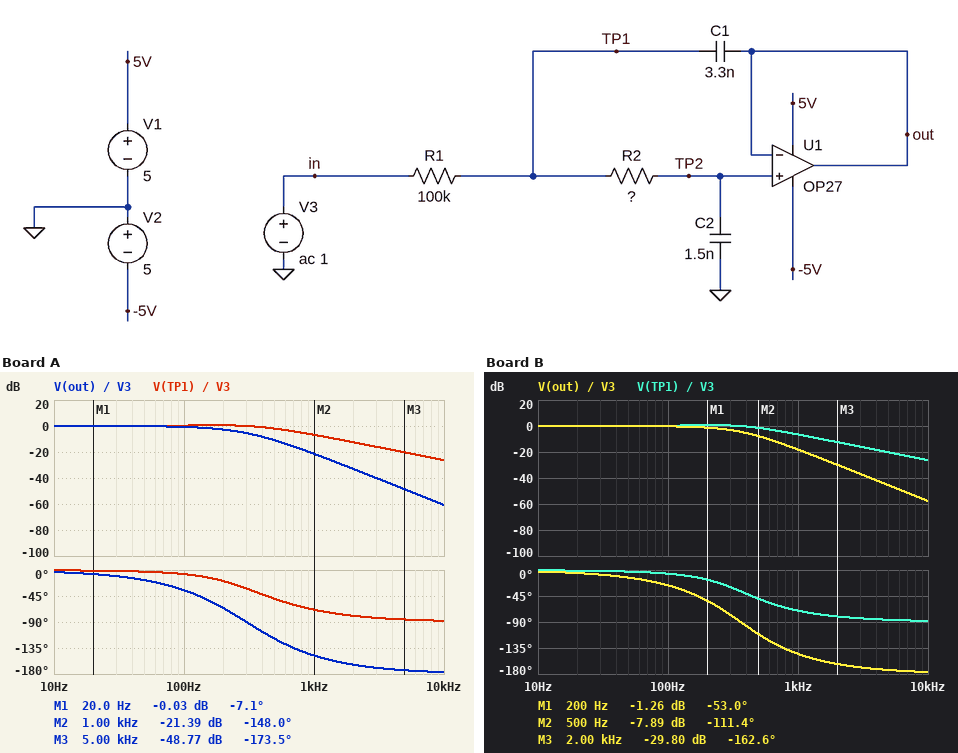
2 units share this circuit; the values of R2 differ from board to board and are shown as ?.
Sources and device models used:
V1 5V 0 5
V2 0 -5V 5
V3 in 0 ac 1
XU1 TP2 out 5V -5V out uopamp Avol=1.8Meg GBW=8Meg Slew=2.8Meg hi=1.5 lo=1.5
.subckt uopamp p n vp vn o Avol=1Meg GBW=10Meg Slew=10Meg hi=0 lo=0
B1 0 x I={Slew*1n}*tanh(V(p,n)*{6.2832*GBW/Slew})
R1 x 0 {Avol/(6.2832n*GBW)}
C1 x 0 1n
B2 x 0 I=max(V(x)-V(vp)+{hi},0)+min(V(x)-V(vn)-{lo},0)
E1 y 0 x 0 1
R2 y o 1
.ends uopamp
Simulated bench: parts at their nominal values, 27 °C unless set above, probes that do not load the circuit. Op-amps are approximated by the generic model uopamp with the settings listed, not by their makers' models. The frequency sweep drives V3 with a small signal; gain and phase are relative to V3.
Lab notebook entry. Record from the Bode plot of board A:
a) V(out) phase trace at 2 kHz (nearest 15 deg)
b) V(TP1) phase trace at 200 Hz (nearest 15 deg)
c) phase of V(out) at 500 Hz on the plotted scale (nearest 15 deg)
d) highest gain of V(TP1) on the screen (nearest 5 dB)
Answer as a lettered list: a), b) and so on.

a) -165 deg
b) -15 deg
c) -120 deg
d) 0 dB
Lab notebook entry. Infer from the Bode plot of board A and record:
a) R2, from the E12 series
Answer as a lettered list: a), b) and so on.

a) 560 kΩ
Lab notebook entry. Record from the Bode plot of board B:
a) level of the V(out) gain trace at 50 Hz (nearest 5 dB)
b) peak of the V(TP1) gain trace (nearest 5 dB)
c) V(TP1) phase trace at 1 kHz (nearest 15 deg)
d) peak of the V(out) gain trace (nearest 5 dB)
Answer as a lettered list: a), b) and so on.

a) 0 dB
b) 0 dB
c) -75 deg
d) 0 dB
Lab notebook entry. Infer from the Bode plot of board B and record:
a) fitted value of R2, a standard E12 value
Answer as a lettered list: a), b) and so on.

a) 390 kΩ
